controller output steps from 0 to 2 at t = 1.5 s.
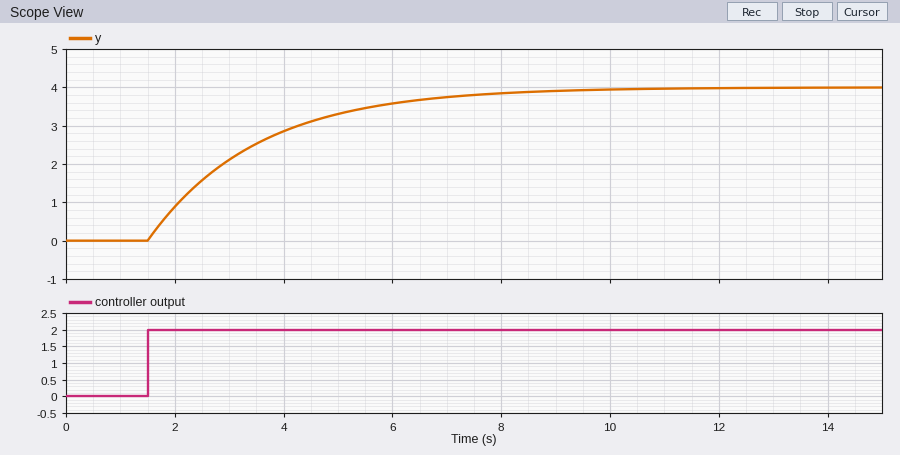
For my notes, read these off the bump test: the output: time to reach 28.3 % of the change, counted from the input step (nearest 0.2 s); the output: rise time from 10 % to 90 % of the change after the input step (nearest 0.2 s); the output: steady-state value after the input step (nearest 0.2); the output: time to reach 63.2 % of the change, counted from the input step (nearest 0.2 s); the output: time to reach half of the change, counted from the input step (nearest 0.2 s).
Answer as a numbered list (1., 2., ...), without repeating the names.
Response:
1. 0.6 s
2. 4.4 s
3. 4.0
4. 2.0 s
5. 1.4 s
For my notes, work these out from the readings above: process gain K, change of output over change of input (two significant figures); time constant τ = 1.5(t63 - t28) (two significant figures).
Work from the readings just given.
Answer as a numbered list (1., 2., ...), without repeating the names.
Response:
1. 2.0
2. 2.1 s
